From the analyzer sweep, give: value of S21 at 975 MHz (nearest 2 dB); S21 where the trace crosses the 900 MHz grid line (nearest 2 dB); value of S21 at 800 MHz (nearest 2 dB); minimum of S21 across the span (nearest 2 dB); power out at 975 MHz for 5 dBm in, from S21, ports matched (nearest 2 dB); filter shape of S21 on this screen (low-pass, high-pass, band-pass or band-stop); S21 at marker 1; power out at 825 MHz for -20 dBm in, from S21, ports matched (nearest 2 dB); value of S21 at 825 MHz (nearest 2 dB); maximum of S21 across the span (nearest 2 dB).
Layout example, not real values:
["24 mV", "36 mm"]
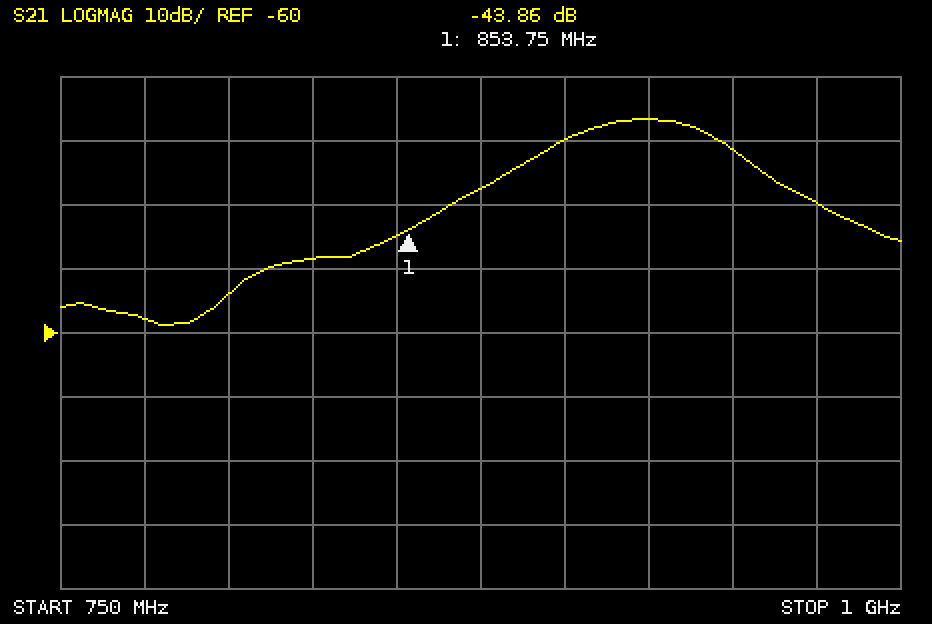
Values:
["-40 dB", "-30 dB", "-54 dB", "-58 dB", "-34 dBm", "band-pass", "-43.86 dB", "-68 dBm", "-48 dB", "-26 dB"]
